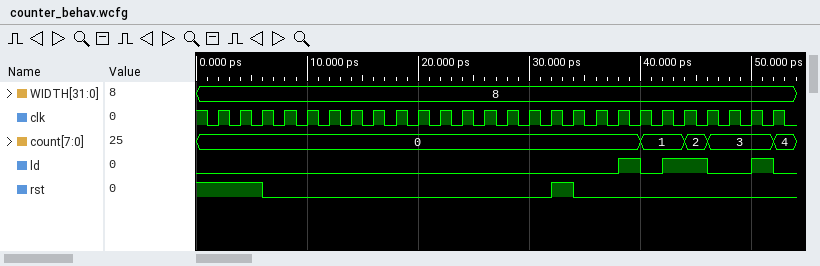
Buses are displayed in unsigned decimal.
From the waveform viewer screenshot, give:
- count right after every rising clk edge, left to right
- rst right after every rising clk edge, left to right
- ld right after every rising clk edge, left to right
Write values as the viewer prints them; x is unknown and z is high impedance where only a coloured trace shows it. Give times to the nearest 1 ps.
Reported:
0, 0, 0, 0, 0, 0, 0, 0, 0, 0, 0, 0, 0, 0, 0, 0, 0, 0, 0, 1, 1, 2, 3, 3, 3, 4
1 1 0 0 0 0 0 0 0 0 0 0 0 0 0 1 0 0 0 0 0 0 0 0 0 0
0 0 0 0 0 0 0 0 0 0 0 0 0 0 0 0 0 0 1 0 1 1 0 0 1 0
